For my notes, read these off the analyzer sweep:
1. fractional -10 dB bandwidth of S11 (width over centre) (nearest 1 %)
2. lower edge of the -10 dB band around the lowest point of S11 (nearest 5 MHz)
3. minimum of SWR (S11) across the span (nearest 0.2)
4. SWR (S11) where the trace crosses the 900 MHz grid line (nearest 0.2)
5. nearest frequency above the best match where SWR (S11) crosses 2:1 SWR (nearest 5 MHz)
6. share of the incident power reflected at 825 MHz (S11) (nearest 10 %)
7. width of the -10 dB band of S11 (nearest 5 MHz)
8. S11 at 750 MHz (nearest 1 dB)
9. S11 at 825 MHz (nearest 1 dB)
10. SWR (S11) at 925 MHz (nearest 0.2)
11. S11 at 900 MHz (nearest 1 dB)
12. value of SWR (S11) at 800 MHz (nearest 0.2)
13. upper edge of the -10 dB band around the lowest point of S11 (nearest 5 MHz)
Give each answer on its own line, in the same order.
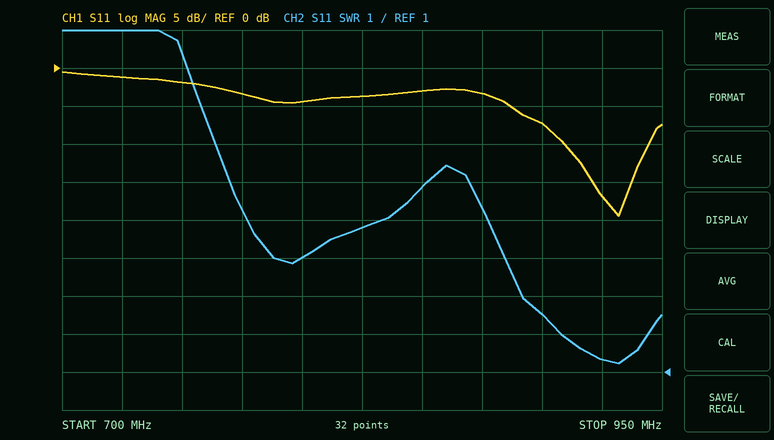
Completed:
4 %
910 MHz
1.2
2.6
945 MHz
40 %
35 MHz
-2 dB
-4 dB
1.4
-7 dB
4.0
945 MHz
